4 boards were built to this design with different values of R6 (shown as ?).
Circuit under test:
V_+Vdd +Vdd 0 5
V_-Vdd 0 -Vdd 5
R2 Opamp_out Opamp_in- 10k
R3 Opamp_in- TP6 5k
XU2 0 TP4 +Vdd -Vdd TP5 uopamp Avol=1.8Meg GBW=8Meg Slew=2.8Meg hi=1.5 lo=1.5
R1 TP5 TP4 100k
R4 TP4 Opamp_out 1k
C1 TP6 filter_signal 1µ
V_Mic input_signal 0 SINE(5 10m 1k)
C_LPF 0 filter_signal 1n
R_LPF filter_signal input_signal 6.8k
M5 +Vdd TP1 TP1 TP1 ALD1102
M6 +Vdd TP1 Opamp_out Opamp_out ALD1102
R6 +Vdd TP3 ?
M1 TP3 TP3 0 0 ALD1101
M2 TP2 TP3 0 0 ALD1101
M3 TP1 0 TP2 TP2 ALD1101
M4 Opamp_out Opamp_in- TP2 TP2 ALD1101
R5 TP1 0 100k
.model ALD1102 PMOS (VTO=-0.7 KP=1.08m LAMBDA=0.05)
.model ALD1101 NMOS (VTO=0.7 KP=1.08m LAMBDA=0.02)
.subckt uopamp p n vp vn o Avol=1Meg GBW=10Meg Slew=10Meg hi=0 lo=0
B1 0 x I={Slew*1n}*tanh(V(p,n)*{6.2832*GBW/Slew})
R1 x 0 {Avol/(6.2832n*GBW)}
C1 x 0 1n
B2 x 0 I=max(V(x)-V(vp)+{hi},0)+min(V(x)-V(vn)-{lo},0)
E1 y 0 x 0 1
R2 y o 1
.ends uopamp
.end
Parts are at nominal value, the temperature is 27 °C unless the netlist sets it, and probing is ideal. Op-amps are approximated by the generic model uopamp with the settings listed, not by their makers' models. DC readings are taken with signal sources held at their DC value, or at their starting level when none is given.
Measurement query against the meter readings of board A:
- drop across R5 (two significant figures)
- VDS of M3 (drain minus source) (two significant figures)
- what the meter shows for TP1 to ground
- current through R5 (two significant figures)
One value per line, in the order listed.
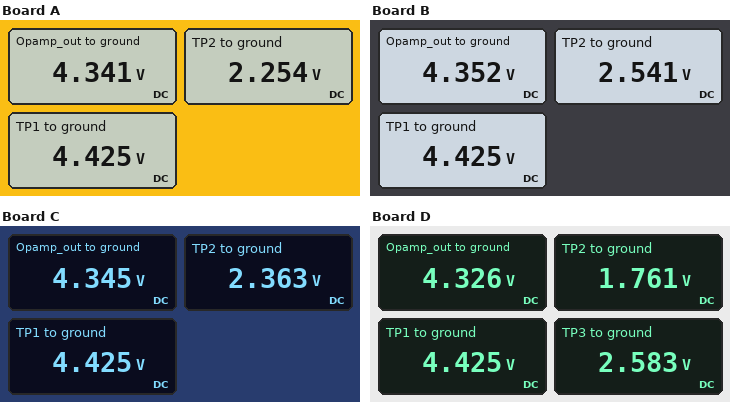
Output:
4.4 V
2.2 V
4.425 V
44 µA
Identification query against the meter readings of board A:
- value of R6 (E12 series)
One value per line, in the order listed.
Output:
2.7 kΩ
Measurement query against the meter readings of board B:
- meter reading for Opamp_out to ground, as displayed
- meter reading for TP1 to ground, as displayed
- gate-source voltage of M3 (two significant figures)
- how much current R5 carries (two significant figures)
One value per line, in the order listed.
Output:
4.352 V
4.425 V
-2.5 V
44 µA
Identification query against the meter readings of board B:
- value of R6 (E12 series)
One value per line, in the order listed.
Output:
4.7 kΩ
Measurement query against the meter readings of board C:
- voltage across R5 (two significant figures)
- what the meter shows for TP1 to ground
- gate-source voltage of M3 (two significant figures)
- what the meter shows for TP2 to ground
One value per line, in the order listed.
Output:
4.4 V
4.425 V
-2.4 V
2.363 V
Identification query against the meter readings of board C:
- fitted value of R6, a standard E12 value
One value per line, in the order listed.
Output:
3.3 kΩ
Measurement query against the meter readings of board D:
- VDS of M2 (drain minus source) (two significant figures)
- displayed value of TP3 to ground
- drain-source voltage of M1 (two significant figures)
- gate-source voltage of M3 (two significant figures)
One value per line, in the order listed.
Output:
1.8 V
2.583 V
2.6 V
-1.8 V
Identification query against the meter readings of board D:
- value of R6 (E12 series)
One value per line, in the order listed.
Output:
1.2 kΩ
